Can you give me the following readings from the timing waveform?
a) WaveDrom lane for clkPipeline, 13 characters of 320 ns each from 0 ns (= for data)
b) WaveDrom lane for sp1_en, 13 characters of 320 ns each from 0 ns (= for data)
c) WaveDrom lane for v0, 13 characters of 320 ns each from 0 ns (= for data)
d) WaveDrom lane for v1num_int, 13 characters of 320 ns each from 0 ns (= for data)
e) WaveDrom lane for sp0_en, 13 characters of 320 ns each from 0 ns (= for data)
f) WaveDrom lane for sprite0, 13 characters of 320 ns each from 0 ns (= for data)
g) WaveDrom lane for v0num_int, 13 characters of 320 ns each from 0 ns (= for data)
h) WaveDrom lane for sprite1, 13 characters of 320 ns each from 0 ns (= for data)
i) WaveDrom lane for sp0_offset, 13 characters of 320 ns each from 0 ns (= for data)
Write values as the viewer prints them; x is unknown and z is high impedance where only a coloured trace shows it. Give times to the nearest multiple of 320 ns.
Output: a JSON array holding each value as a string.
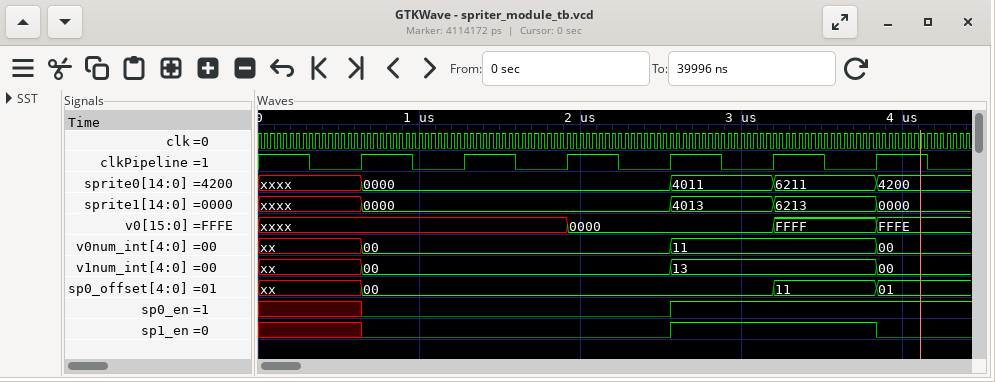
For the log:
["{name: 'clkPipeline', wave: '1010101010101'}", "{name: 'sp1_en', wave: 'x.0.....1...0'}", "{name: 'v0', wave: 'x.....=...=.=', data: '0000 FFFF FFFE'}", "{name: 'v1num_int', wave: 'x.=.....=...=', data: '00 13 00'}", "{name: 'sp0_en', wave: 'x.0.....1....'}", "{name: 'sprite0', wave: 'x.=.....=.=.=', data: '0000 4011 6211 4200'}", "{name: 'v0num_int', wave: 'x.=.....=...=', data: '00 11 00'}", "{name: 'sprite1', wave: 'x.=.....=.=.=', data: '0000 4013 6213 0000'}", "{name: 'sp0_offset', wave: 'x.=.......=.=', data: '00 11 01'}"]
